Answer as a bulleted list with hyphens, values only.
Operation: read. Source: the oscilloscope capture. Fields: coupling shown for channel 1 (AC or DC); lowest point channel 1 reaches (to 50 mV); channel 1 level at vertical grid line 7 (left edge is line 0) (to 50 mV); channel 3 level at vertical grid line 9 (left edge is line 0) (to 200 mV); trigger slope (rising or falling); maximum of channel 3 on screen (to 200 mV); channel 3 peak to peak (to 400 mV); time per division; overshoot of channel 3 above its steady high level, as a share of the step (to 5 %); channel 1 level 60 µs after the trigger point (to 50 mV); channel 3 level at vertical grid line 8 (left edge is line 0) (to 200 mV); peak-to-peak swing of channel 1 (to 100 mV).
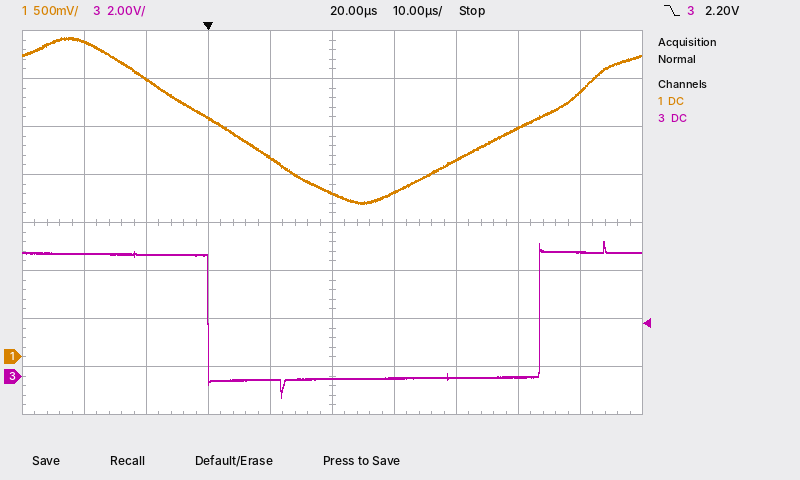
- DC
- 1.60 V
- 2.05 V
- 5.2 V
- falling
- 5.6 V
- 6.4 V
- 10 µs
- 10 %
- 2.75 V
- 0.0 V
- 1.70 V
